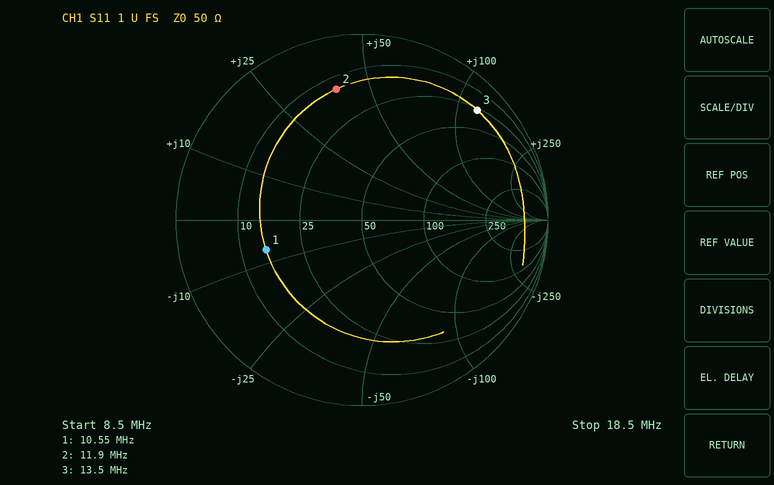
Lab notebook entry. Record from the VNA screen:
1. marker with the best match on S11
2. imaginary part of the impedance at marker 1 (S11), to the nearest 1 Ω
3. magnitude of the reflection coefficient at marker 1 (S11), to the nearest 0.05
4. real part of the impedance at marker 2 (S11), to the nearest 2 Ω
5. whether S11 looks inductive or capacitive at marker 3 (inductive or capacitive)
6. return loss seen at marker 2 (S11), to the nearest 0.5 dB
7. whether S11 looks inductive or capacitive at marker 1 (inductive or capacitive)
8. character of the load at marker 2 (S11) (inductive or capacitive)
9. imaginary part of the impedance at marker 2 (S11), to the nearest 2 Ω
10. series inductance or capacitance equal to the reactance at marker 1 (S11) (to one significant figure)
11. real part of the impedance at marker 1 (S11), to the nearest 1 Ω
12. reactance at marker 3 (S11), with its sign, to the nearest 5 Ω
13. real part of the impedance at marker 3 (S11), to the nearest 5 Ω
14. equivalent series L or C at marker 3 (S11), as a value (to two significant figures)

marker 1
-7 Ω
0.55
14 Ω
inductive
3.0 dB
capacitive
inductive
+40 Ω
2 nF
15 Ω
+120 Ω
25 Ω
1.4 µH
